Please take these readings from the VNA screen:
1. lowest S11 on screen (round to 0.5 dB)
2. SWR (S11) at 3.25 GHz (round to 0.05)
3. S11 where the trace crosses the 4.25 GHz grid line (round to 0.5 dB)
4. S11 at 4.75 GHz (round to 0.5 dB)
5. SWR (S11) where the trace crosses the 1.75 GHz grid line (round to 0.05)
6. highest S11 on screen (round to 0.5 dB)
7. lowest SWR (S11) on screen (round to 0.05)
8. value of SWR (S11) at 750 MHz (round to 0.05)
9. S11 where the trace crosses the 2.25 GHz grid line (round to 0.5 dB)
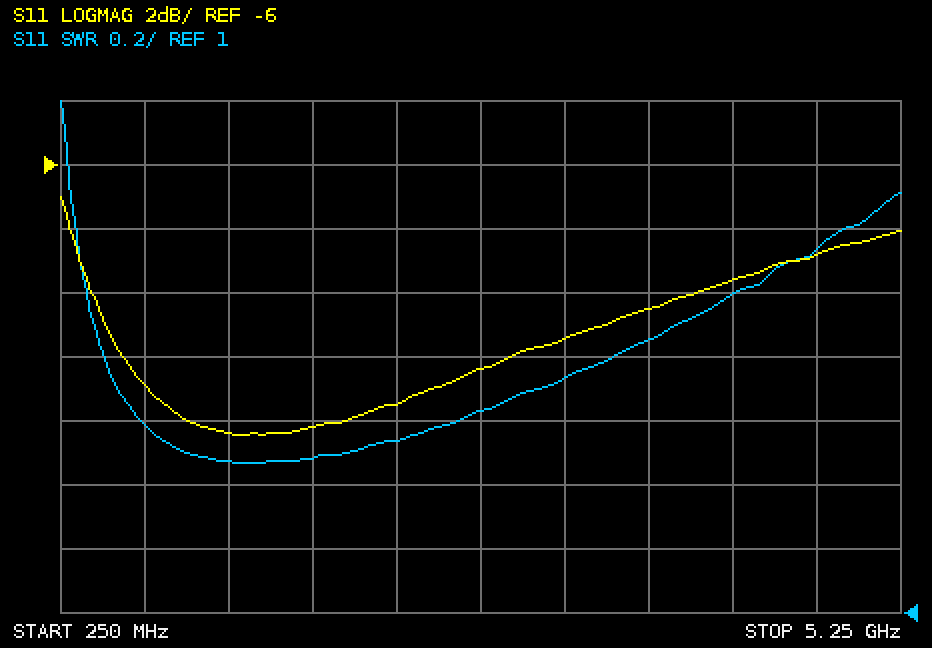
-14.5 dB
1.75
-9.5 dB
-9.0 dB
1.50
-7.0 dB
1.45
1.60
-13.5 dB
